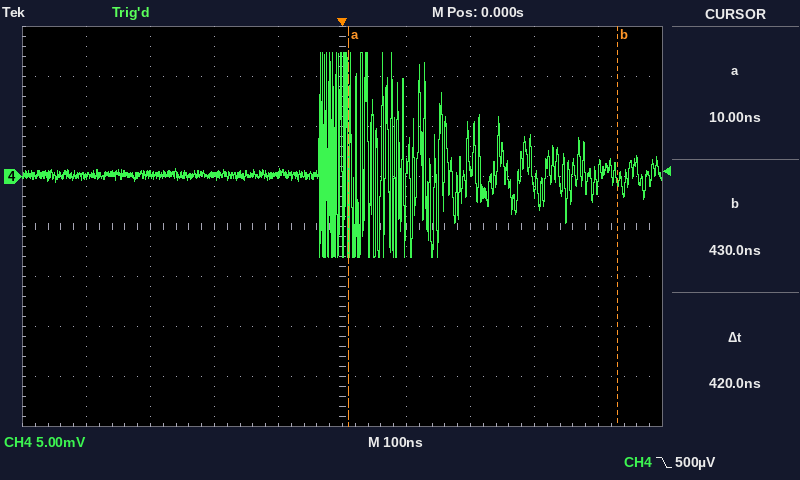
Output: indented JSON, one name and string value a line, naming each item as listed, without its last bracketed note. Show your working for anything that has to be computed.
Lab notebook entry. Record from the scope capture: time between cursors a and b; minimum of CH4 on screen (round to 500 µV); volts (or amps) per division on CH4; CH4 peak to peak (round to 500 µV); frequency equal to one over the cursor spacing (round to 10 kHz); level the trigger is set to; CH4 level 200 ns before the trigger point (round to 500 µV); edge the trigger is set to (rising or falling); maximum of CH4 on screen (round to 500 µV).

{
  "time between cursors a and b": "420 ns",
  "minimum of CH4 on screen": "-8.0 mV",
  "volts (or amps) per division on CH4": "5 mV",
  "CH4 peak to peak": "12.5 mV − (-8.0 mV) = 20.5 mV",
  "frequency equal to one over the cursor spacing": "1 / 420 ns ≈ 2.38 MHz",
  "level the trigger is set to": "500 µV",
  "CH4 level 200 ns before the trigger point": "0.0 mV",
  "edge the trigger is set to": "falling",
  "maximum of CH4 on screen": "12.5 mV"
}
